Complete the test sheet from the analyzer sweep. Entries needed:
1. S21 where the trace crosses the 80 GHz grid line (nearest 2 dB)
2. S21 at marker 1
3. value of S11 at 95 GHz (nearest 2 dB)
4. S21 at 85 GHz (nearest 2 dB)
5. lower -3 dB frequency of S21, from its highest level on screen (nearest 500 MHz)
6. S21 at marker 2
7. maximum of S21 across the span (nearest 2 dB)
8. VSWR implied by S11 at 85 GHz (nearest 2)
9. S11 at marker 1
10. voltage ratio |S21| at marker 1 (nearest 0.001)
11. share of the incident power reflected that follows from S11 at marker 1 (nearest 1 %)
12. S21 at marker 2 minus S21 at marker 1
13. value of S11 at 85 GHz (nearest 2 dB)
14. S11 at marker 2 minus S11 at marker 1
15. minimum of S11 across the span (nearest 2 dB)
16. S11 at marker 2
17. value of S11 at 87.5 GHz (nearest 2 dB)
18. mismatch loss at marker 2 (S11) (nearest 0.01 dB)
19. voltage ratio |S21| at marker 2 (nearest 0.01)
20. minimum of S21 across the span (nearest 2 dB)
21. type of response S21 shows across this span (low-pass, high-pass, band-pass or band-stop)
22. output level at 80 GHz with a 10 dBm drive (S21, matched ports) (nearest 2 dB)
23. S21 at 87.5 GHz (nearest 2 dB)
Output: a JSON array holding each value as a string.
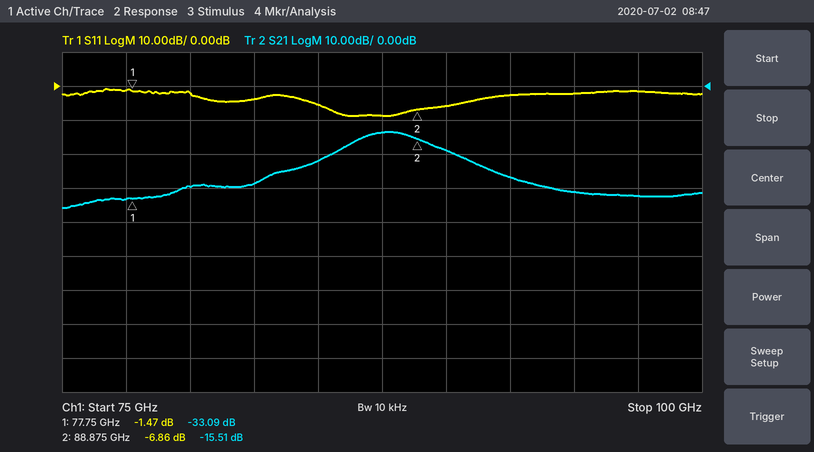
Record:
["-30 dB", "-33.09 dB", "-2 dB", "-22 dB", "86.5 GHz", "-15.51 dB", "-14 dB", "4", "-1.47 dB", "0.022", "71 %", "17.58 dB", "-6 dB", "-5.39 dB", "-8 dB", "-6.86 dB", "-8 dB", "1.00 dB", "0.17", "-36 dB", "band-pass", "-20 dBm", "-14 dB"]
